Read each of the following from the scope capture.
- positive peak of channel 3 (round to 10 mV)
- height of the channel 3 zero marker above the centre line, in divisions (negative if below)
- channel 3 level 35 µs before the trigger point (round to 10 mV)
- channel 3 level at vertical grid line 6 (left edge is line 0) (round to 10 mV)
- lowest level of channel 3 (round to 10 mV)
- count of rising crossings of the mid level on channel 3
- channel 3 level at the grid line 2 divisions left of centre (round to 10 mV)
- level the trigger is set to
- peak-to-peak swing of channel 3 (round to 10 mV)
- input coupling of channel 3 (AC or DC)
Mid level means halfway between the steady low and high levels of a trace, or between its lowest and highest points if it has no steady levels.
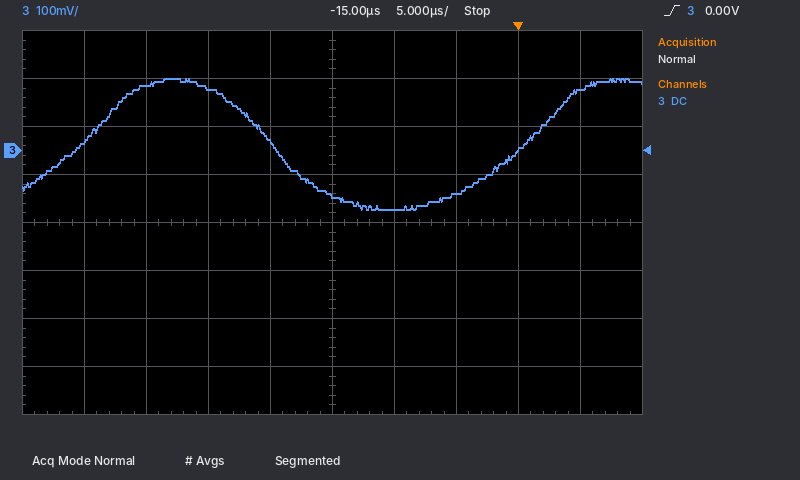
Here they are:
150 mV
+1.5 div
20 mV
-120 mV
-120 mV
2
130 mV
0.00 V
270 mV
DC
